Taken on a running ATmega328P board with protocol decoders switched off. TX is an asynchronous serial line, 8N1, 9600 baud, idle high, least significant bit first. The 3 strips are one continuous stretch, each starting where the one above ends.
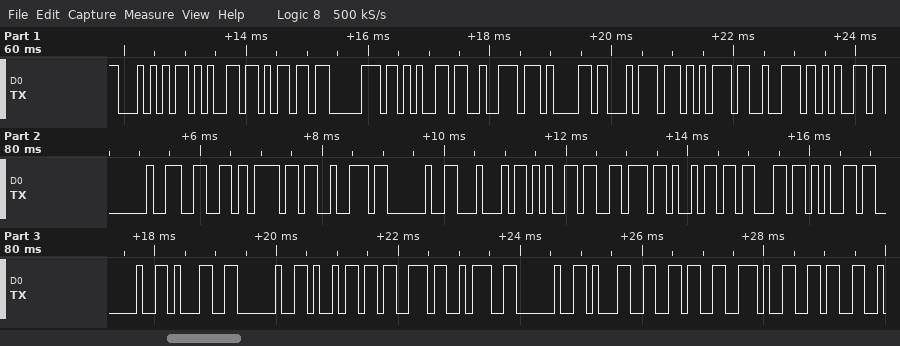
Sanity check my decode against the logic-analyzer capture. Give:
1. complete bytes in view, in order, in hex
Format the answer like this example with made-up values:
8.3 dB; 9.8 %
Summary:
54 65 6D 70 65 72 61 74 75 72 65 20 66 6F 72 20 44 65 76 69 63 65 20 31 20 69 73 3A 20 31 36 2E 36
